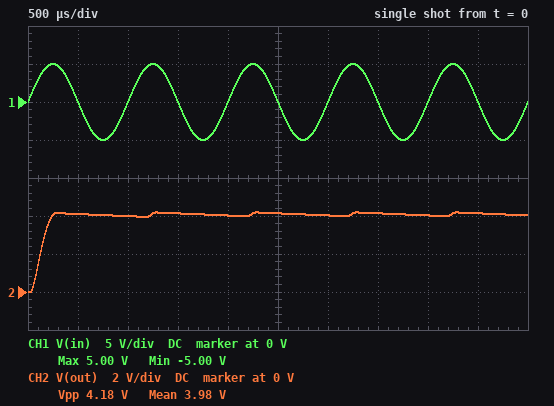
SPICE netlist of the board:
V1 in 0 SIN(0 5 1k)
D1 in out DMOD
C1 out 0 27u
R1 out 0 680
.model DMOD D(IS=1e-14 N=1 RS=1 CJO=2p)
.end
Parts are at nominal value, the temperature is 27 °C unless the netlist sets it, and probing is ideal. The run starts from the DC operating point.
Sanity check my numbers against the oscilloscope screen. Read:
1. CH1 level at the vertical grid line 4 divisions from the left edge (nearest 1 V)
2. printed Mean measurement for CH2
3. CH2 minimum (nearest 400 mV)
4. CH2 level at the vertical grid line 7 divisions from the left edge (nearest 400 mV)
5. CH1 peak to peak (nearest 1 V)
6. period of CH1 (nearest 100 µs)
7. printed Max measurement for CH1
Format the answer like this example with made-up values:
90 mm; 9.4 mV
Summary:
0 V; 3.98 V; 0 V; 4.0 V; 10 V; 1.0 ms; 5.00 V
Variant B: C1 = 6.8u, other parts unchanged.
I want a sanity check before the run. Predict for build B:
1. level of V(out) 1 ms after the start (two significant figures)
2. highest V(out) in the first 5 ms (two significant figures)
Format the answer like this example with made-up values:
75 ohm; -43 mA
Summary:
3.6 V; 4.3 V
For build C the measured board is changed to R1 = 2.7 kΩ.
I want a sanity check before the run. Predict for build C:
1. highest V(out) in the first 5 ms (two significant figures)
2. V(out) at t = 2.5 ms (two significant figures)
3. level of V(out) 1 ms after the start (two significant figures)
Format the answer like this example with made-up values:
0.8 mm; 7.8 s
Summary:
4.2 V; 4.2 V; 4.1 V
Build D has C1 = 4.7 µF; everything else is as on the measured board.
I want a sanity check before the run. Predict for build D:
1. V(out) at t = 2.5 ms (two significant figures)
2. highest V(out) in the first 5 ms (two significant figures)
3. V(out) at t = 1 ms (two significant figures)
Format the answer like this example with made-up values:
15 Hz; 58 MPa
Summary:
4.0 V; 4.3 V; 3.4 V
